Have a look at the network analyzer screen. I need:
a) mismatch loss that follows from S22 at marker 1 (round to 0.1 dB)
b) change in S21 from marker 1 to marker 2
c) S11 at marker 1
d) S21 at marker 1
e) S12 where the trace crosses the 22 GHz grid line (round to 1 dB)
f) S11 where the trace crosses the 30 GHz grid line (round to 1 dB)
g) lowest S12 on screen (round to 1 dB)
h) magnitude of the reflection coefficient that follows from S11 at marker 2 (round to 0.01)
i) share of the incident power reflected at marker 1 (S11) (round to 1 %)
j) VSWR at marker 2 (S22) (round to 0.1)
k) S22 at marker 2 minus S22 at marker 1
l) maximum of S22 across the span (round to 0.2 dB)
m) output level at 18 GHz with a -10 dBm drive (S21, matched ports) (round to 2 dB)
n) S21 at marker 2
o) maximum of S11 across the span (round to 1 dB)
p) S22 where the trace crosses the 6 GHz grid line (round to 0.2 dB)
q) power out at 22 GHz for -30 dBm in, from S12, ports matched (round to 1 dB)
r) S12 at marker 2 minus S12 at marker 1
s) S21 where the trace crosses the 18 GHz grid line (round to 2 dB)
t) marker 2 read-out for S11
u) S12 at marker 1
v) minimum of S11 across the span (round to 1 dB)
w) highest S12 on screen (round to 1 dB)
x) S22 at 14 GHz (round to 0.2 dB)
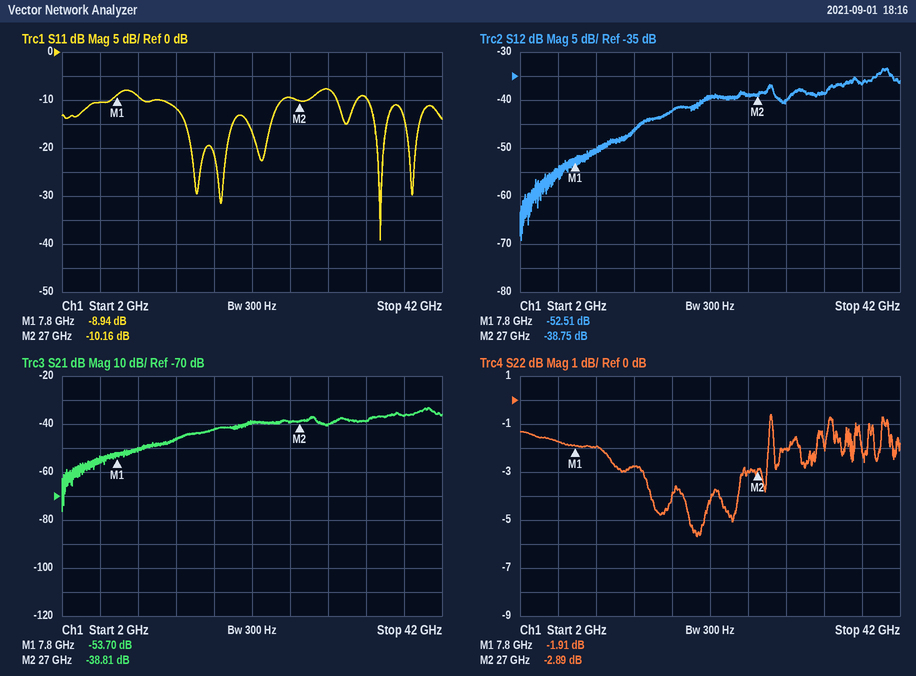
4.5 dB
14.89 dB
-8.94 dB
-53.70 dB
-39 dB
-8 dB
-69 dB
0.31
13 %
6.1
-0.98 dB
-0.6 dB
-52 dBm
-38.81 dB
-8 dB
-1.8 dB
-69 dBm
13.76 dB
-42 dB
-10.16 dB
-52.51 dB
-39 dB
-33 dB
-2.8 dB
